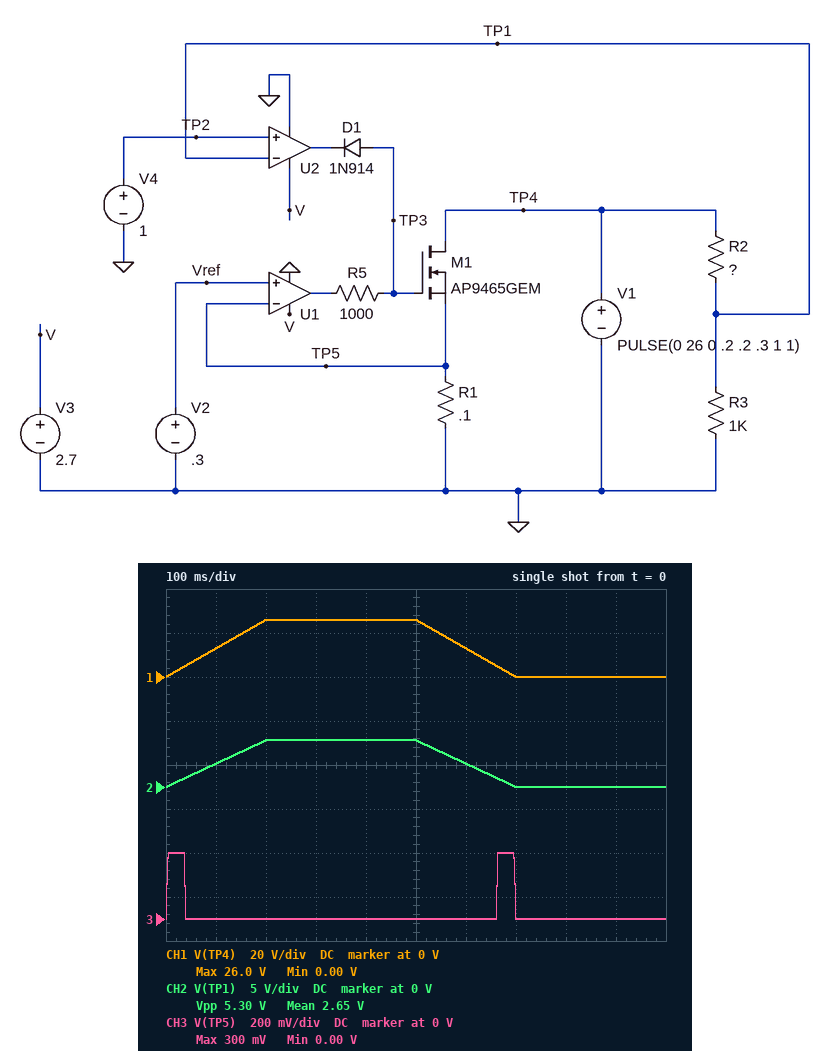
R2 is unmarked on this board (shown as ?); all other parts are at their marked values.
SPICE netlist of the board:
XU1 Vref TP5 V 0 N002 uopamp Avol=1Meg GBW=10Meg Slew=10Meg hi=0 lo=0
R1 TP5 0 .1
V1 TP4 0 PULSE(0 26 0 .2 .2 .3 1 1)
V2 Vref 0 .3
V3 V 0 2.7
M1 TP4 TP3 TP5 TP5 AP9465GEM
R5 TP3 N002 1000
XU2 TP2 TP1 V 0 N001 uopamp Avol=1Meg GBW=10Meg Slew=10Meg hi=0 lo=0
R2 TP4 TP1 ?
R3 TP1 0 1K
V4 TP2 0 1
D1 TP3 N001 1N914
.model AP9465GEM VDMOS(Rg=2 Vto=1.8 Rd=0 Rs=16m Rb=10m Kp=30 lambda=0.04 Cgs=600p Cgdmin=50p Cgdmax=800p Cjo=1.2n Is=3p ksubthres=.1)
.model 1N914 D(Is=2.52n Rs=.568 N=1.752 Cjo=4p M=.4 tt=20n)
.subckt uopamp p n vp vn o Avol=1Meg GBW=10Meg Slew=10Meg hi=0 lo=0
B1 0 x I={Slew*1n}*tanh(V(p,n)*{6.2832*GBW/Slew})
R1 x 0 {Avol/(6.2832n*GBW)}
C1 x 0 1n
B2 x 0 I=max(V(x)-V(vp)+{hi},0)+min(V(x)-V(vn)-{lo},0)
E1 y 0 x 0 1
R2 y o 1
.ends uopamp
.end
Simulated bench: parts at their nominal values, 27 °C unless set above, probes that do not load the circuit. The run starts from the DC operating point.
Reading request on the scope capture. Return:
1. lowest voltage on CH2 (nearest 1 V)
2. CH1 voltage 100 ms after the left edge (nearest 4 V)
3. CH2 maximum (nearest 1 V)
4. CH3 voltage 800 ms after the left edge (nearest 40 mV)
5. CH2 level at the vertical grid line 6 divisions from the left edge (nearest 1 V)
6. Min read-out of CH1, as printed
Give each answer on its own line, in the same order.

0 V
12 V
5 V
0 V
3 V
0.00 V
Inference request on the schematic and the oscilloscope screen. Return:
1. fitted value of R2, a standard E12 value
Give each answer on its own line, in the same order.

3.9 kΩ
